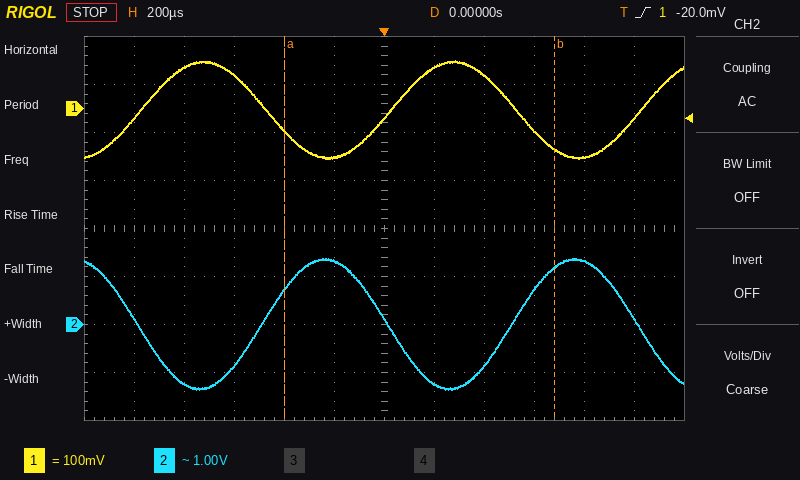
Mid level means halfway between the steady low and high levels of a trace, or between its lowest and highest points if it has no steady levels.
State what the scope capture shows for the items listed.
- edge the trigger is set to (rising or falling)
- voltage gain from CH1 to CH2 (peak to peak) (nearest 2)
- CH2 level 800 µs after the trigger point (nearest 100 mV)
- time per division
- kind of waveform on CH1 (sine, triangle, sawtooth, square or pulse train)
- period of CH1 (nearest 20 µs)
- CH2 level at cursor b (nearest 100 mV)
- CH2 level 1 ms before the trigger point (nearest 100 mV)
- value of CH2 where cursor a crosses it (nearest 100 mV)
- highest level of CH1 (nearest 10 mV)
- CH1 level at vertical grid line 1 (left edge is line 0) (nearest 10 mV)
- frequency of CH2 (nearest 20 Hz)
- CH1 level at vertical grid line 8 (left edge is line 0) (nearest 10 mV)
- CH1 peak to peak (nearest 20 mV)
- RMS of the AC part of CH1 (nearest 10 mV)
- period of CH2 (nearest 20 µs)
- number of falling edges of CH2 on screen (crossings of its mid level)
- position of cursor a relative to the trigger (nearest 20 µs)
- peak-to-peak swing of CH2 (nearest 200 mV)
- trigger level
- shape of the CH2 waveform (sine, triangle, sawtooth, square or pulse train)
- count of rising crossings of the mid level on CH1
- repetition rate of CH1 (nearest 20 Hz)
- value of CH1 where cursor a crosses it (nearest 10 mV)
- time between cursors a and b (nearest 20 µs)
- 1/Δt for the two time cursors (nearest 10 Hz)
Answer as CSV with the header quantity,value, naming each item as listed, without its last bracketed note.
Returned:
quantity,value
edge the trigger is set to,rising
voltage gain from CH1 to CH2 (peak to peak),14
CH2 level 800 µs after the trigger point,1.3 V
time per division,200 µs
kind of waveform on CH1,sine
period of CH1,1.00 ms
CH2 level at cursor b,1.2 V
CH2 level 1 ms before the trigger point,100 mV
value of CH2 where cursor a crosses it,700 mV
highest level of CH1,100 mV
CH1 level at vertical grid line 1 (left edge is line 0),-20 mV
frequency of CH2,1.00 kHz
CH1 level at vertical grid line 8 (left edge is line 0),70 mV
CH1 peak to peak,200 mV
RMS of the AC part of CH1,70 mV
period of CH2,1.00 ms
number of falling edges of CH2 on screen,3
position of cursor a relative to the trigger,-400 µs
peak-to-peak swing of CH2,2.8 V
trigger level,-20.0 mV
shape of the CH2 waveform,sine
count of rising crossings of the mid level on CH1,3
repetition rate of CH1,1.00 kHz
value of CH1 where cursor a crosses it,-50 mV
time between cursors a and b,1.08 ms
1/Δt for the two time cursors,930 Hz
